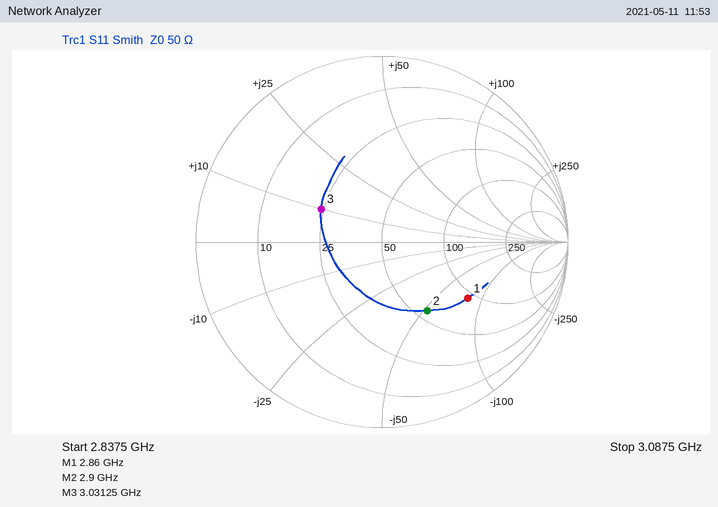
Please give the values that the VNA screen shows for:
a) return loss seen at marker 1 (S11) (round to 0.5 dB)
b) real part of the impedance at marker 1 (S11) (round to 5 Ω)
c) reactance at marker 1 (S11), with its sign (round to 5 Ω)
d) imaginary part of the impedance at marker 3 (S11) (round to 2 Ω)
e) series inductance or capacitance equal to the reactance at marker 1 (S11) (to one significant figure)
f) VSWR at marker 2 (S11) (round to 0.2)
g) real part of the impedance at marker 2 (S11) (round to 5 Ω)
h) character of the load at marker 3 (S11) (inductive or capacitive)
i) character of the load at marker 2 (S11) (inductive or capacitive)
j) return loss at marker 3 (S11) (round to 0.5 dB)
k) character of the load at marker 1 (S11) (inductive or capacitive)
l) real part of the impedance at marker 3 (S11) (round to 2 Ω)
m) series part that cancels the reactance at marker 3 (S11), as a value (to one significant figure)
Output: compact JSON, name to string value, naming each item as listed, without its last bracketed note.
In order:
{"return loss seen at marker 1 (S11)": "5.0 dB", "real part of the impedance at marker 1 (S11)": "90 Ω", "reactance at marker 1 (S11), with its sign": "-80 Ω", "imaginary part of the impedance at marker 3 (S11)": "+10 Ω", "series inductance or capacitance equal to the reactance at marker 1 (S11)": "700 fF", "VSWR at marker 2 (S11)": "2.6", "real part of the impedance at marker 2 (S11)": "55 Ω", "character of the load at marker 3 (S11)": "inductive", "character of the load at marker 2 (S11)": "capacitive", "return loss at marker 3 (S11)": "8.5 dB", "character of the load at marker 1 (S11)": "capacitive", "real part of the impedance at marker 3 (S11)": "24 Ω", "series part that cancels the reactance at marker 3 (S11), as a value": "5 pF"}
